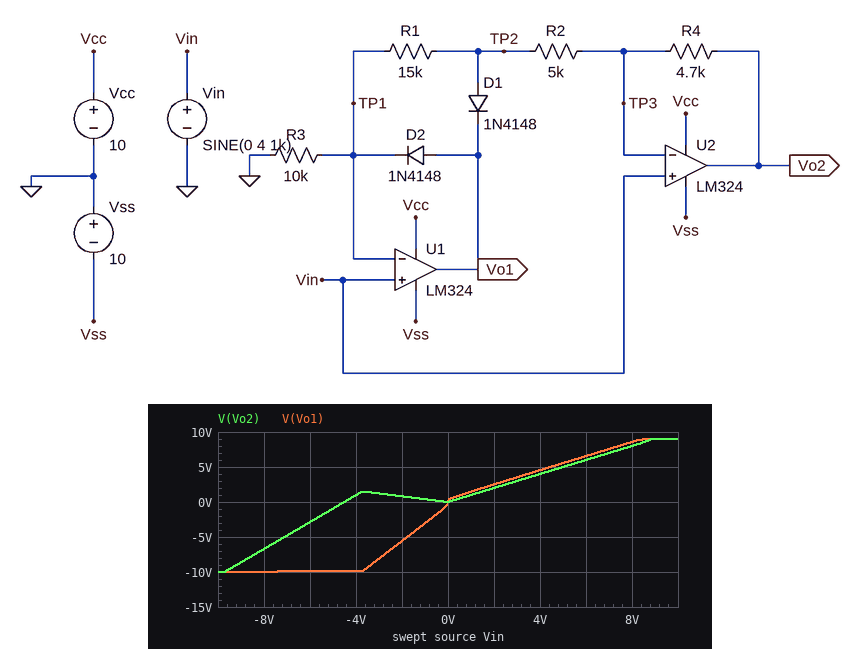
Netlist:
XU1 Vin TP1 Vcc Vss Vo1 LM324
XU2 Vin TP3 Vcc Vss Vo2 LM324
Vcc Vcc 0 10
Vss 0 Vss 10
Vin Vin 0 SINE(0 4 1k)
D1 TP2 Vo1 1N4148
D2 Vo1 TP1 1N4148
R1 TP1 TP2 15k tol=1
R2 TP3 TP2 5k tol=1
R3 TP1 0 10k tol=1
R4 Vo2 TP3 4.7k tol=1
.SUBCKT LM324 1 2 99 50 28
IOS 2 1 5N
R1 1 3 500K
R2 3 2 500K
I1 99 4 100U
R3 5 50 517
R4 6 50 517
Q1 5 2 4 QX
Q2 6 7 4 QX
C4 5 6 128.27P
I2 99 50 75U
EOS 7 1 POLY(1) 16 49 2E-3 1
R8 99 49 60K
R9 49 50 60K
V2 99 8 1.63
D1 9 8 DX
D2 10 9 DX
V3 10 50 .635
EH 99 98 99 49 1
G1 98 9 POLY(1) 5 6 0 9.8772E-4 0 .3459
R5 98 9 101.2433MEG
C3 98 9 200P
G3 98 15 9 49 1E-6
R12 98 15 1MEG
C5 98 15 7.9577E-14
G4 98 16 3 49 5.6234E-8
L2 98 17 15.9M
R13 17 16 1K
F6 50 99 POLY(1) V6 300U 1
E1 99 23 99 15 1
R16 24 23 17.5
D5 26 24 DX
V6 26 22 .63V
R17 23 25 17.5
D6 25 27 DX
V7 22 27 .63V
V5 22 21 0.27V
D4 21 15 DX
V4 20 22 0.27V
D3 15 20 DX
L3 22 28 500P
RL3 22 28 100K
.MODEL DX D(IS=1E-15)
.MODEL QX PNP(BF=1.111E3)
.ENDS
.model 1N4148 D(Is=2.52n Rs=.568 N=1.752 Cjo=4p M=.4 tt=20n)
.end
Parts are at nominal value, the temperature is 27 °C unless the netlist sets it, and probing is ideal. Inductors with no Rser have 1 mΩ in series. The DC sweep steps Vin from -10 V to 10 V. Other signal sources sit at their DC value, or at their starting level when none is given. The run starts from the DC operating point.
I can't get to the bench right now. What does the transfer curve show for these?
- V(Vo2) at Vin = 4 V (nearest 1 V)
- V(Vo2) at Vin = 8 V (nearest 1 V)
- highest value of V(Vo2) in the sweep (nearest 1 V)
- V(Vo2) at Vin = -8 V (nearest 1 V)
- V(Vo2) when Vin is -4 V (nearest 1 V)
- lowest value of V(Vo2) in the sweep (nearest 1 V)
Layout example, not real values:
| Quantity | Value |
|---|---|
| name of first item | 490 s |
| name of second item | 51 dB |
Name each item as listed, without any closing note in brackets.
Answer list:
| Quantity | Value |
|---|---|
| V(Vo2) at Vin = 4 V | 4 V |
| V(Vo2) at Vin = 8 V | 8 V |
| highest value of V(Vo2) in the sweep | 9 V |
| V(Vo2) at Vin = -8 V | -7 V |
| V(Vo2) when Vin is -4 V | 1 V |
| lowest value of V(Vo2) in the sweep | -10 V |
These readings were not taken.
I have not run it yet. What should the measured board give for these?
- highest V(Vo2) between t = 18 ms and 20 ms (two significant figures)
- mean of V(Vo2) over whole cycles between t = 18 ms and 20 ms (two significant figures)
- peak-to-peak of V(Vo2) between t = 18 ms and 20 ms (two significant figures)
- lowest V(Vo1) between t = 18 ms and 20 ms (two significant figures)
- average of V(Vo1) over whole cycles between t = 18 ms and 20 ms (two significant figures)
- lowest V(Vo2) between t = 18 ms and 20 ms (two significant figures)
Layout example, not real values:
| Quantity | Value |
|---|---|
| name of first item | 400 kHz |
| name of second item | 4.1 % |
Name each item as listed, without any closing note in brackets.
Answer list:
| Quantity | Value |
|---|---|
| highest V(Vo2) between t = 18 ms and 20 ms | 4.0 V |
| mean of V(Vo2) over whole cycles between t = 18 ms and 20 ms | 1.7 V |
| peak-to-peak of V(Vo2) between t = 18 ms and 20 ms | 4.1 V |
| lowest V(Vo1) between t = 18 ms and 20 ms | -9.9 V |
| average of V(Vo1) over whole cycles between t = 18 ms and 20 ms | -1.9 V |
| lowest V(Vo2) between t = 18 ms and 20 ms | -110 mV |
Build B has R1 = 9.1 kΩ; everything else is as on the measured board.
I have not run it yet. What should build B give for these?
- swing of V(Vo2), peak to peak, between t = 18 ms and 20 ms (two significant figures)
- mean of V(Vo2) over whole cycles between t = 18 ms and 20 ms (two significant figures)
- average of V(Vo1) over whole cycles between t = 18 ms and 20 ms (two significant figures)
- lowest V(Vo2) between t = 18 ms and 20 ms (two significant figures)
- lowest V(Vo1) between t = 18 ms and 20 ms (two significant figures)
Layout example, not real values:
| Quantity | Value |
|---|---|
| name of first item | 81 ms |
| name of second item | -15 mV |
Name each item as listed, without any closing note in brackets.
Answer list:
| Quantity | Value |
|---|---|
| swing of V(Vo2), peak to peak, between t = 18 ms and 20 ms | 4.6 V |
| mean of V(Vo2) over whole cycles between t = 18 ms and 20 ms | 1.1 V |
| average of V(Vo1) over whole cycles between t = 18 ms and 20 ms | -1.2 V |
| lowest V(Vo2) between t = 18 ms and 20 ms | -580 mV |
| lowest V(Vo1) between t = 18 ms and 20 ms | -8.2 V |
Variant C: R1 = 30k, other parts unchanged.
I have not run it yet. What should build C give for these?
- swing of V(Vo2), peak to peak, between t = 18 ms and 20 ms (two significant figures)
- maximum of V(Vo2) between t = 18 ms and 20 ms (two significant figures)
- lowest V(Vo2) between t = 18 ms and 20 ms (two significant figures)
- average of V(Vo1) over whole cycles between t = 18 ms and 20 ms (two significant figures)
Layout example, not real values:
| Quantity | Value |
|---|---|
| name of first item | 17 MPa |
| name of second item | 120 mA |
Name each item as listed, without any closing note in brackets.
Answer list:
| Quantity | Value |
|---|---|
| swing of V(Vo2), peak to peak, between t = 18 ms and 20 ms | 4.3 V |
| maximum of V(Vo2) between t = 18 ms and 20 ms | 4.2 V |
| lowest V(Vo2) between t = 18 ms and 20 ms | -96 mV |
| average of V(Vo1) over whole cycles between t = 18 ms and 20 ms | -2.5 V |
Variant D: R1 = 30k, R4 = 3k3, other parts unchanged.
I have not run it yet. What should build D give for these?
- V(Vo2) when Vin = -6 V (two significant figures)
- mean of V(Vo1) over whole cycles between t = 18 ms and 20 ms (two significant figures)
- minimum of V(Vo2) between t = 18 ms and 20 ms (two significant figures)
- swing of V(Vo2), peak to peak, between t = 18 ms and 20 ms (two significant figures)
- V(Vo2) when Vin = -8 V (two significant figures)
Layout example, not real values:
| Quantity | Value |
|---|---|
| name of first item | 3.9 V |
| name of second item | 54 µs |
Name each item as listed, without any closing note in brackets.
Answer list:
| Quantity | Value |
|---|---|
| V(Vo2) when Vin = -6 V | -3.8 V |
| mean of V(Vo1) over whole cycles between t = 18 ms and 20 ms | -2.5 V |
| minimum of V(Vo2) between t = 18 ms and 20 ms | -490 mV |
| swing of V(Vo2), peak to peak, between t = 18 ms and 20 ms | 4.5 V |
| V(Vo2) when Vin = -8 V | -7.1 V |
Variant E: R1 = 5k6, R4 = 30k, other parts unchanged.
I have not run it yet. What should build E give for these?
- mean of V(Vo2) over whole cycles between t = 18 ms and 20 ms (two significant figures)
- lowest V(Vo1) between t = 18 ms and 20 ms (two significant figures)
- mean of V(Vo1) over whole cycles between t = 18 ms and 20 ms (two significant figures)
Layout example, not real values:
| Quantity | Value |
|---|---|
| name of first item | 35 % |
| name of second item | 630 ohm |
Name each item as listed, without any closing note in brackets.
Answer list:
| Quantity | Value |
|---|---|
| mean of V(Vo2) over whole cycles between t = 18 ms and 20 ms | 4.2 V |
| lowest V(Vo1) between t = 18 ms and 20 ms | -6.8 V |
| mean of V(Vo1) over whole cycles between t = 18 ms and 20 ms | -730 mV |
